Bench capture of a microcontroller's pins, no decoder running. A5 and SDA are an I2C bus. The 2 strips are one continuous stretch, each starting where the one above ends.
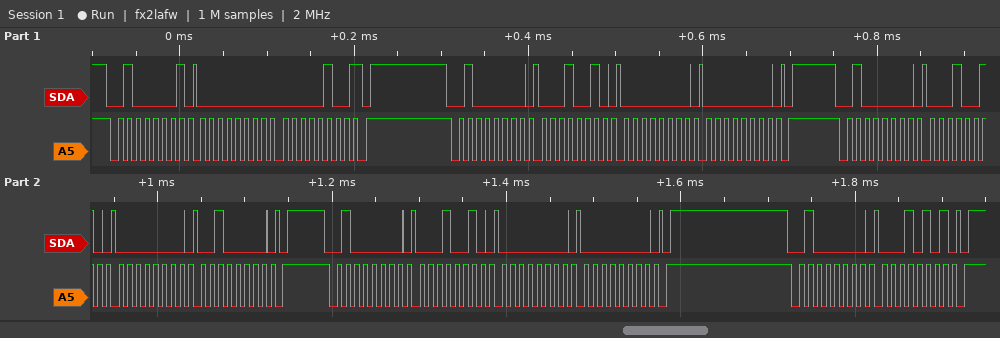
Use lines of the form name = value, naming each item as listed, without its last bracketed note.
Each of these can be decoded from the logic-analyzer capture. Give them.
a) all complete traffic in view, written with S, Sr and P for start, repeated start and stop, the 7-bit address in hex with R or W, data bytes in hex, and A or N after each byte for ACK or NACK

all complete traffic in view, written with S, Sr and P for start, repeated start and stop, the 7-bit address in hex with R or W, data bytes in hex, and A or N after each byte for ACK or NACK = S 20R A 00 A 04 N P S 20W A 12 A 00 A 00 A P S 20W A 12 A 00 A 20 A P S 20W A 12 A 00 A 00 A P S 20W A 15 A P
